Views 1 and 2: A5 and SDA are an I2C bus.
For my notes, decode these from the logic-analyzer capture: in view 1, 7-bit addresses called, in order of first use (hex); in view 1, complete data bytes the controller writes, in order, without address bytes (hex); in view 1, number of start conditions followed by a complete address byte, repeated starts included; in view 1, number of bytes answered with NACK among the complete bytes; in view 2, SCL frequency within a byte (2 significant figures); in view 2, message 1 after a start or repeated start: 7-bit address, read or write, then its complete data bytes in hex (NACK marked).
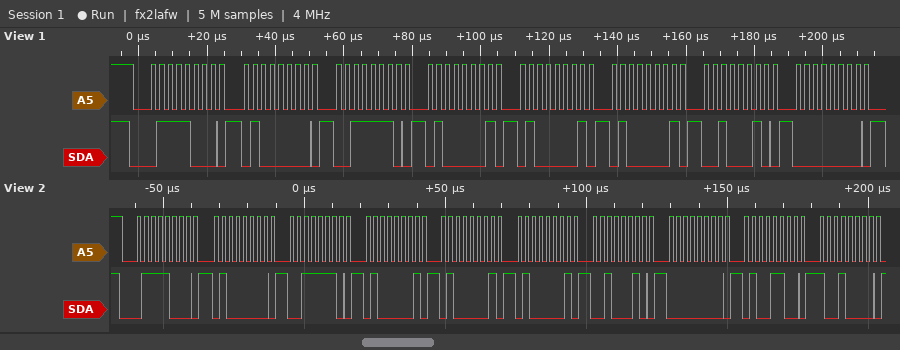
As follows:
0x3C
40 3E 41 41 41 22 00
1
0
400 kHz
0x3C write: 40 3E 41 41 41 22 00 4C 90
